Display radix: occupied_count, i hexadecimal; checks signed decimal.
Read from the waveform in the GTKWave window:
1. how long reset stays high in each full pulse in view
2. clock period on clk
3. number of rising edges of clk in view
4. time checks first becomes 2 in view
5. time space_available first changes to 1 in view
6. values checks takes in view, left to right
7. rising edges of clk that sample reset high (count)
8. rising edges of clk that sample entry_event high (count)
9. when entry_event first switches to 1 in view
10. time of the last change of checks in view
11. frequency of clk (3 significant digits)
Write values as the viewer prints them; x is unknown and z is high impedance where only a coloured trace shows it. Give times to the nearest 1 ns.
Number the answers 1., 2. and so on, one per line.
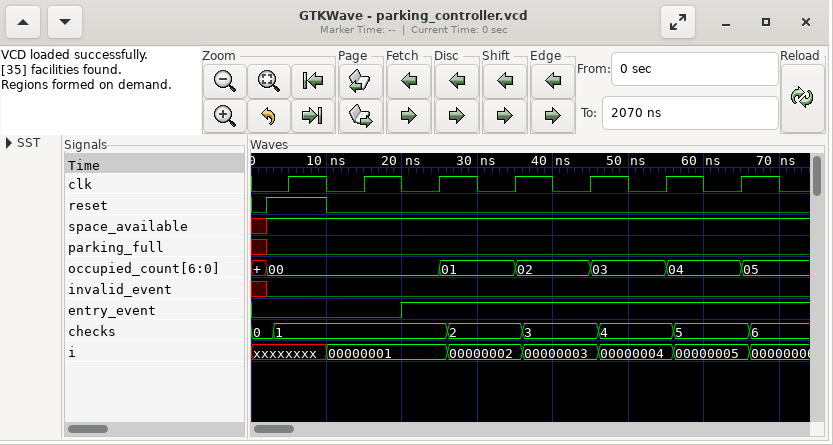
1. 8 ns
2. 10 ns
3. 7
4. 26 ns
5. 2 ns
6. 0, 1, 2, 3, 4, 5, 6
7. 1
8. 5
9. 20 ns
10. 66 ns
11. 100 MHz
